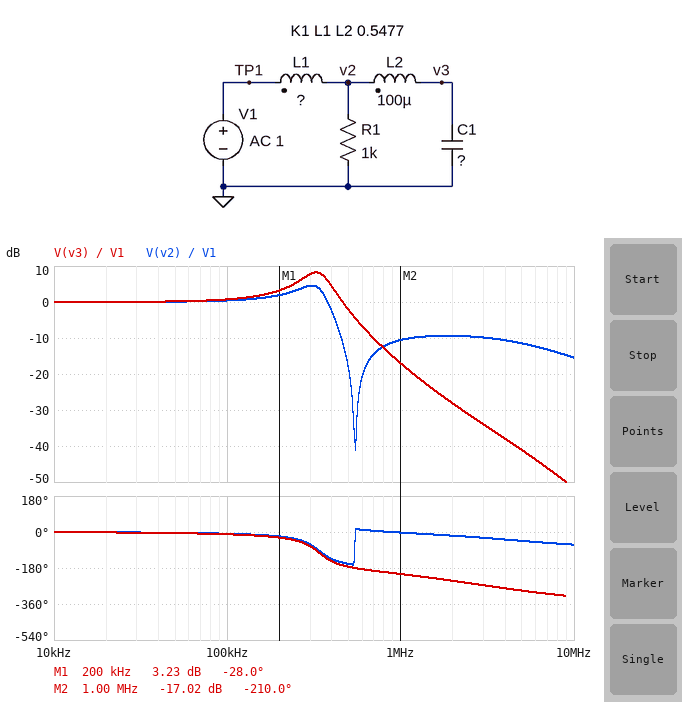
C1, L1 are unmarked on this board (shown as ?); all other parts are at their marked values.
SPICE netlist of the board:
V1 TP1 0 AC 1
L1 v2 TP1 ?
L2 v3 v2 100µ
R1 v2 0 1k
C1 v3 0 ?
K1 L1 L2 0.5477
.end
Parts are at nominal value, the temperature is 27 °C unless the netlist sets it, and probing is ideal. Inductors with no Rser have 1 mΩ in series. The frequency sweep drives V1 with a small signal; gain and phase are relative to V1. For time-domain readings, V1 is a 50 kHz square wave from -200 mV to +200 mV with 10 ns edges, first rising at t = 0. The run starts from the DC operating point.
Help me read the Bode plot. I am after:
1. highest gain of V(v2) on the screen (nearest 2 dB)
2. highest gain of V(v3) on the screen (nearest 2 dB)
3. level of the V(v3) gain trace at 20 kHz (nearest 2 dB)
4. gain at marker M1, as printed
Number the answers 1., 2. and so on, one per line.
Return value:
1. 4 dB
2. 8 dB
3. 0 dB
4. 3.23 dB
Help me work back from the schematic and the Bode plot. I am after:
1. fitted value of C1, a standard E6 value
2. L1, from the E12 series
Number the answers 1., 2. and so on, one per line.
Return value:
1. 470 pF
2. 220 µH
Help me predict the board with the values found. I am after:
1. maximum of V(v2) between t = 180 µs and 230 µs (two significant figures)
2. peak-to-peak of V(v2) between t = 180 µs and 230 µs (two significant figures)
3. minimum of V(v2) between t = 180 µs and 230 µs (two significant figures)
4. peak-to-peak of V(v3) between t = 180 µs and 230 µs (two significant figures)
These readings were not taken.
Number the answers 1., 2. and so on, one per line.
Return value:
1. 330 mV
2. 670 mV
3. -330 mV
4. 830 mV
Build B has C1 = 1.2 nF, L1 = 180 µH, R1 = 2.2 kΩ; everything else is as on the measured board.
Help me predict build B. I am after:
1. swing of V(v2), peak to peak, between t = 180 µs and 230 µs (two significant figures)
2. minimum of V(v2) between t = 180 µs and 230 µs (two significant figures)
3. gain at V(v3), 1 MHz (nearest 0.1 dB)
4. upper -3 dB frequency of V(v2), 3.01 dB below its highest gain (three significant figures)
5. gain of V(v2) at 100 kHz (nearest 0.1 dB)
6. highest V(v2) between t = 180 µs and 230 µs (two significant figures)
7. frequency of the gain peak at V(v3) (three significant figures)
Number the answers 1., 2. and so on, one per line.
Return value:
1. 730 mV
2. -370 mV
3. -25.5 dB
4. 231 kHz
5. 1.2 dB
6. 370 mV
7. 222 kHz
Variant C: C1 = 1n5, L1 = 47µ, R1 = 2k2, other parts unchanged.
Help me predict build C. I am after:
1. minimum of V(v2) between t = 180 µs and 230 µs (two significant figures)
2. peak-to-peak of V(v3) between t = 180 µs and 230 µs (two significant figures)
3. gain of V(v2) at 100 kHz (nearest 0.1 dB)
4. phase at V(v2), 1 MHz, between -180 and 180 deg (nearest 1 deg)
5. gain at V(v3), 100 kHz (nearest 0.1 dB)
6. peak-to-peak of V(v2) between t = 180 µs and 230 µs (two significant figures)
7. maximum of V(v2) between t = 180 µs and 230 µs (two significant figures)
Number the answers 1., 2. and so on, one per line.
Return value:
1. -310 mV
2. 1.0 V
3. 0.5 dB
4. -2 deg
5. 1.2 dB
6. 630 mV
7. 310 mV
